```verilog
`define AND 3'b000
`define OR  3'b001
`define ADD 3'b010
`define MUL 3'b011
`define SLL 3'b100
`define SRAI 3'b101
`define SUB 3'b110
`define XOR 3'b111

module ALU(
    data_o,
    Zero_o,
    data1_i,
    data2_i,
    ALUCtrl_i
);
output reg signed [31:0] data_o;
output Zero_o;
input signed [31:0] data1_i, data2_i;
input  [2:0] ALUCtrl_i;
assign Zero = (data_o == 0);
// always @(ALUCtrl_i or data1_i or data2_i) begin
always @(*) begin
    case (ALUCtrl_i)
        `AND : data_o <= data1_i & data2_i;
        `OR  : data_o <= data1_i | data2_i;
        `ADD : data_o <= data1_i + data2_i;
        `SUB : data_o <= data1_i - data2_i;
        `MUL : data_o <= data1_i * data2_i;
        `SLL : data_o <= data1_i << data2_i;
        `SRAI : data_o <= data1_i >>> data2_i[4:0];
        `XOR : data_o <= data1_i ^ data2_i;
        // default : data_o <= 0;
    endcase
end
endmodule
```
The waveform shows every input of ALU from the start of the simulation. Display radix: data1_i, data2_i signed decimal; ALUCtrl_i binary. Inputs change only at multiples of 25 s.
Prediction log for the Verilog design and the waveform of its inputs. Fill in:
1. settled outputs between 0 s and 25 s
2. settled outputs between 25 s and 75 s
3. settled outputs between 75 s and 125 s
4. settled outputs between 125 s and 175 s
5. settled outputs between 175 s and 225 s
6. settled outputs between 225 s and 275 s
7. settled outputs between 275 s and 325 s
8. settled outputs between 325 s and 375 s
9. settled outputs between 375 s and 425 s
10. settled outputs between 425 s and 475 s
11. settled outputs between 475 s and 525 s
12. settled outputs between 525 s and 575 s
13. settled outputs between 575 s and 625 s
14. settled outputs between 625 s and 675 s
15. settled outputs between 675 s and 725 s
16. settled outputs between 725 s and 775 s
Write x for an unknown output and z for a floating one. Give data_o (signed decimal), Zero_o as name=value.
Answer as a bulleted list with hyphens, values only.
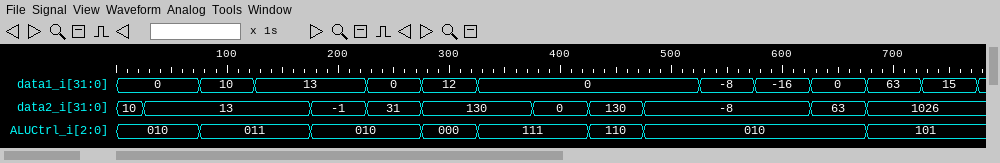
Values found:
- data_o=10, Zero_o=z
- data_o=13, Zero_o=z
- data_o=130, Zero_o=z
- data_o=169, Zero_o=z
- data_o=12, Zero_o=z
- data_o=31, Zero_o=z
- data_o=0, Zero_o=z
- data_o=130, Zero_o=z
- data_o=0, Zero_o=z
- data_o=-130, Zero_o=z
- data_o=-8, Zero_o=z
- data_o=-16, Zero_o=z
- data_o=-24, Zero_o=z
- data_o=63, Zero_o=z
- data_o=15, Zero_o=z
- data_o=3, Zero_o=z
